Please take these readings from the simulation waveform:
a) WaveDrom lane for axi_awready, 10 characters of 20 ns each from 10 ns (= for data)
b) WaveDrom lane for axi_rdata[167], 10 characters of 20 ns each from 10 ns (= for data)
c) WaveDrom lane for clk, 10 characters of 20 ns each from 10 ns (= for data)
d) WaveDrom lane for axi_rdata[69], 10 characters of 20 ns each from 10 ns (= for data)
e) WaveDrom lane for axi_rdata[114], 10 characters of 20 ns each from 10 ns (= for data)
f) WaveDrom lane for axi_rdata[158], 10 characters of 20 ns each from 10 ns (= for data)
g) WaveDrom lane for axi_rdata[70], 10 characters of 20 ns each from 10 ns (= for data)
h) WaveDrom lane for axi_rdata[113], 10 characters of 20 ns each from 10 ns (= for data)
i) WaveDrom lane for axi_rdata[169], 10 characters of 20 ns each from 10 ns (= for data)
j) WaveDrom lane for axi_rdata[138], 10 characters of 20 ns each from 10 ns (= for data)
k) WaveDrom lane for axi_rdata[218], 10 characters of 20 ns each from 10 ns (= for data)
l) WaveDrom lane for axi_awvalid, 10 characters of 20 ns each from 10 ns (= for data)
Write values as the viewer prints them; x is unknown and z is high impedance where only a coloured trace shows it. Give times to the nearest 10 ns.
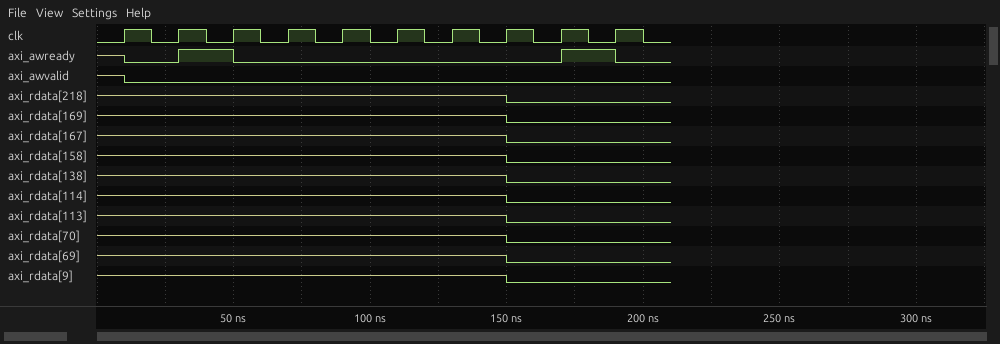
{name: 'axi_awready', wave: '010.....10'}
{name: 'axi_rdata[167]', wave: 'z......0..'}
{name: 'clk', wave: 'p.........'}
{name: 'axi_rdata[69]', wave: 'z......0..'}
{name: 'axi_rdata[114]', wave: 'z......0..'}
{name: 'axi_rdata[158]', wave: 'z......0..'}
{name: 'axi_rdata[70]', wave: 'z......0..'}
{name: 'axi_rdata[113]', wave: 'z......0..'}
{name: 'axi_rdata[169]', wave: 'z......0..'}
{name: 'axi_rdata[138]', wave: 'z......0..'}
{name: 'axi_rdata[218]', wave: 'z......0..'}
{name: 'axi_awvalid', wave: '0.........'}
